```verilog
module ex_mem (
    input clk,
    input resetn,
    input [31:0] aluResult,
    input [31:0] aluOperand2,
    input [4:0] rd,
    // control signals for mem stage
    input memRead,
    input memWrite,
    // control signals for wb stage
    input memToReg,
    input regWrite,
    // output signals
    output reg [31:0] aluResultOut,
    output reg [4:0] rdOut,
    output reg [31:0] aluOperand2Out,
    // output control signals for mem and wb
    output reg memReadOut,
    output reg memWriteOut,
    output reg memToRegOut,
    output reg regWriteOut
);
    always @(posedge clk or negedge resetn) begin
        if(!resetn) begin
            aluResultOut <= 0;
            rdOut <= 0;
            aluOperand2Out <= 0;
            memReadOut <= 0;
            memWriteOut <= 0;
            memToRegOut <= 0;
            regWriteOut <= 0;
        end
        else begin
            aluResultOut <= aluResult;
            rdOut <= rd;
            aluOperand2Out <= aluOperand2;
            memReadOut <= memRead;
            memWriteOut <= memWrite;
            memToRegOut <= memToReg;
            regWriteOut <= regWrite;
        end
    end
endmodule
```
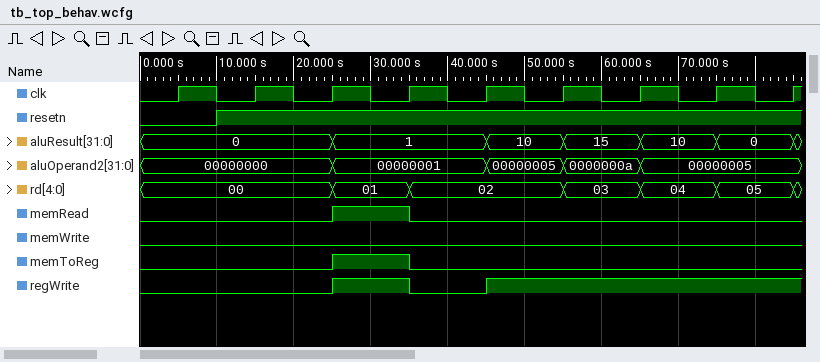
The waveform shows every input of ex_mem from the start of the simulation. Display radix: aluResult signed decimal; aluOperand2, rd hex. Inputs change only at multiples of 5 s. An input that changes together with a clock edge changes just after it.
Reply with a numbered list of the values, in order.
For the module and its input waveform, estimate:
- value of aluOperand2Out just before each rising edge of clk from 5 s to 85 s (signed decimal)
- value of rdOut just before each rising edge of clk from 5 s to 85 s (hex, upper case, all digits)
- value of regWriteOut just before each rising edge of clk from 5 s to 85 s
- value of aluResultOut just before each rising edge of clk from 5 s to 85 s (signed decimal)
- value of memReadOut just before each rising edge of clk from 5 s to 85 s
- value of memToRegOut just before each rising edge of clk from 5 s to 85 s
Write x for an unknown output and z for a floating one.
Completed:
1. 0, 0, 0, 0, 1, 1, 5, 10, 5
2. 00, 00, 00, 00, 01, 02, 02, 03, 04
3. 0 0 0 0 1 0 1 1 1
4. 0, 0, 0, 0, 1, 1, 10, 15, 10
5. 0 0 0 0 1 0 0 0 0
6. 0 0 0 0 1 0 0 0 0
